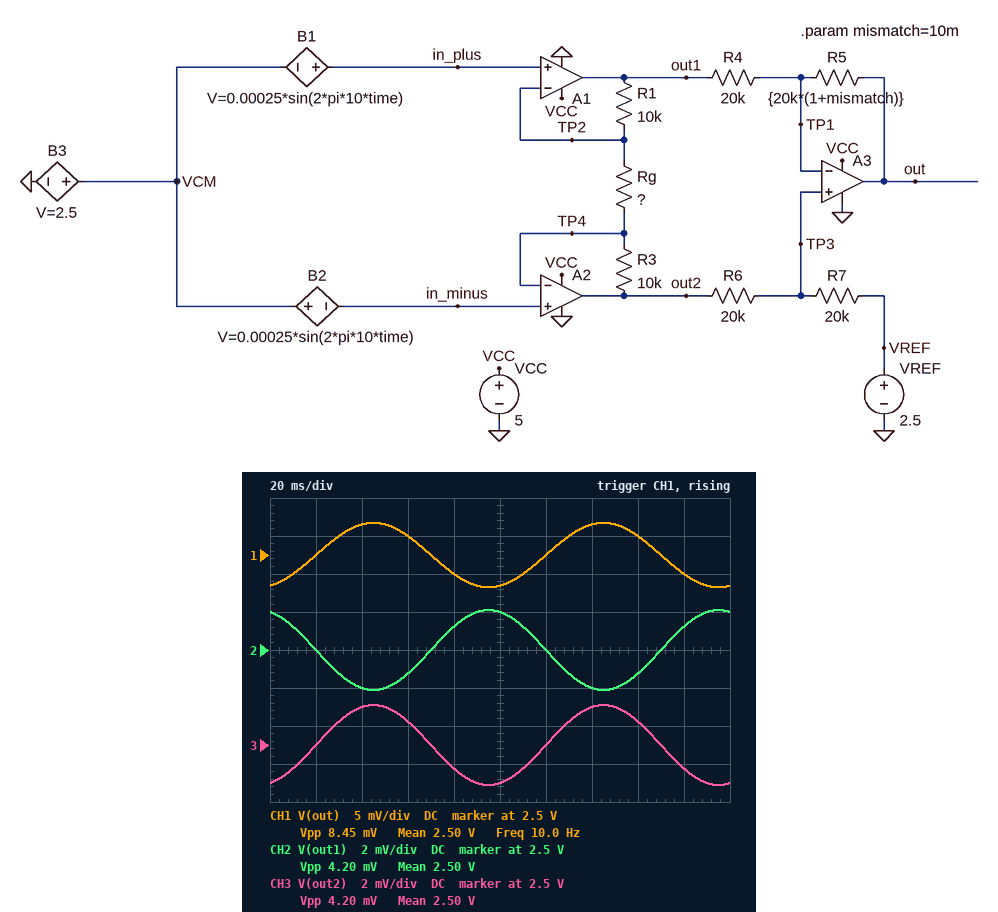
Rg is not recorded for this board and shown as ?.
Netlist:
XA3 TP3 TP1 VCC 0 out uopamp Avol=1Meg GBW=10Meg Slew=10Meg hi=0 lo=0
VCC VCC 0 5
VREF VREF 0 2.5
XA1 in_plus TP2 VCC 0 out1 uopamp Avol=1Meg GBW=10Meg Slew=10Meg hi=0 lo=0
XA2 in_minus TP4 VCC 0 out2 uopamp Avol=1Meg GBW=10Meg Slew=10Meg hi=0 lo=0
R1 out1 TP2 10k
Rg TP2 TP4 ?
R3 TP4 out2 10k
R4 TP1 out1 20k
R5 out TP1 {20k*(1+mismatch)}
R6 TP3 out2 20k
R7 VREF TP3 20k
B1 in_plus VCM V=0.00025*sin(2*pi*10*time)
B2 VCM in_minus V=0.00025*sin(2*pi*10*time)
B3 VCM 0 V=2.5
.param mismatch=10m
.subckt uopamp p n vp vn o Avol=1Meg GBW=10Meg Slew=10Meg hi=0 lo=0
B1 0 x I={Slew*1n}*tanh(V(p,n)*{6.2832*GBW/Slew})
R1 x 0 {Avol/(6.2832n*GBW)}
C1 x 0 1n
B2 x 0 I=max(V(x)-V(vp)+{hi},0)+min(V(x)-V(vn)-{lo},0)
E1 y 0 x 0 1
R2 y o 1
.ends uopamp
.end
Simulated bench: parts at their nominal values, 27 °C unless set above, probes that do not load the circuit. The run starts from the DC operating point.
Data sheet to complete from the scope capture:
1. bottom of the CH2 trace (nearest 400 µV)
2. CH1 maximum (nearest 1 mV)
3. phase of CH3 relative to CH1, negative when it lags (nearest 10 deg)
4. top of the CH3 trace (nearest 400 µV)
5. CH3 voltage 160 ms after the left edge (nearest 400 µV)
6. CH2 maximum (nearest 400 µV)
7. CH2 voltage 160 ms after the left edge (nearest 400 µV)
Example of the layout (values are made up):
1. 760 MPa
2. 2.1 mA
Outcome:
1. 2.4980 V
2. 2.504 V
3. 0 deg
4. 2.5020 V
5. 2.5012 V
6. 2.5020 V
7. 2.4988 V
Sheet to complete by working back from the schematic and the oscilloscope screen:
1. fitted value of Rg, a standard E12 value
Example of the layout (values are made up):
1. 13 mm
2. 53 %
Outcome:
1. 2.7 kΩ
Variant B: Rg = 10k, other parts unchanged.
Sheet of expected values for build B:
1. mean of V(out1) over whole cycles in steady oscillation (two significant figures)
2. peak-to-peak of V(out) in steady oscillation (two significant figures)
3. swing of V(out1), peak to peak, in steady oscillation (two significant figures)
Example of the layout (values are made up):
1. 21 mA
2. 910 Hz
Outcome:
1. 2.5 V
2. 3.0 mV
3. 1.5 mV
